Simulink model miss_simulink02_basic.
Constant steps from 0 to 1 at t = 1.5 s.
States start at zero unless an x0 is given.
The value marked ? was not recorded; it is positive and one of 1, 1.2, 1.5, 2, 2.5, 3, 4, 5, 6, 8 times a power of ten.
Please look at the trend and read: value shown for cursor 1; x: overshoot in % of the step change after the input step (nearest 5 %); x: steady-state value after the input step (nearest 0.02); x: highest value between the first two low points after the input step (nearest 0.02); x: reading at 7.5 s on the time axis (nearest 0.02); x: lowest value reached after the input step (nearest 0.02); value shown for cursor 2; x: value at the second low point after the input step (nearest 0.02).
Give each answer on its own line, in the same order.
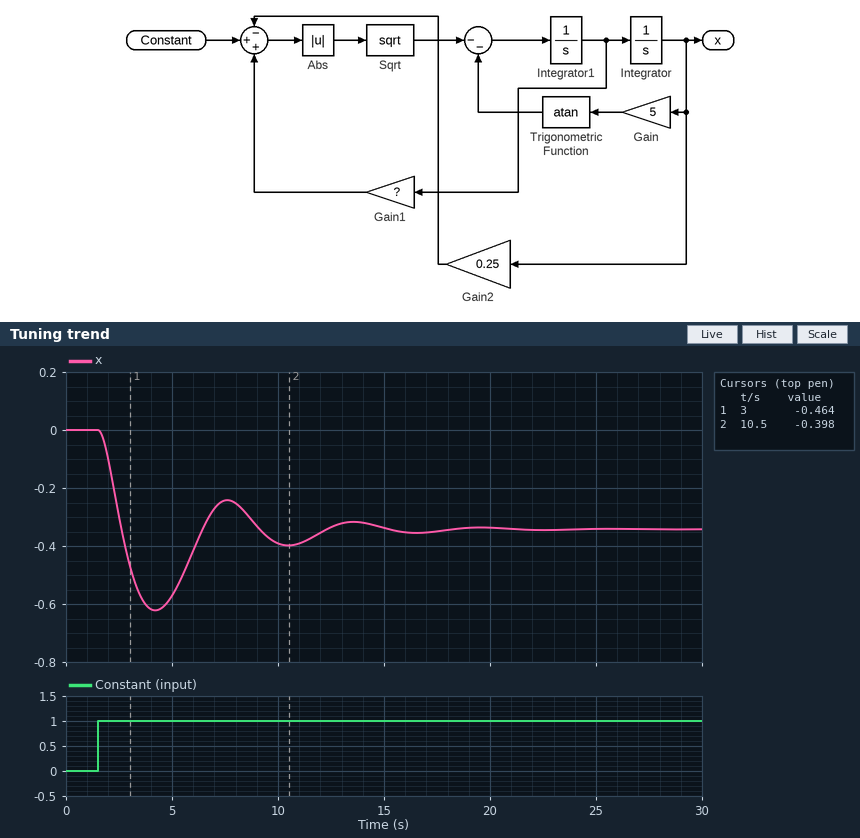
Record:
-0.464
80 %
-0.34
-0.24
-0.24
-0.62
-0.398
-0.40
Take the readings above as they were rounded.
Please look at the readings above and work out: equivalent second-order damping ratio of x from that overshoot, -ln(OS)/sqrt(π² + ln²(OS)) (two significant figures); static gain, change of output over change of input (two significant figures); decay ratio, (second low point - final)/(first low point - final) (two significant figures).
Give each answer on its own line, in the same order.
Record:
0.071
-0.34
0.21
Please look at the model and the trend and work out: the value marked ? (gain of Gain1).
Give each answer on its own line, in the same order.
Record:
1
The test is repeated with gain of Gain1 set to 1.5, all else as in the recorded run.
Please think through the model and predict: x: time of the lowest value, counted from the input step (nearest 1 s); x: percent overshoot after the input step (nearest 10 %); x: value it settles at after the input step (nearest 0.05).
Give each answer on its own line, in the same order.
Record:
3 s
50 %
-0.35
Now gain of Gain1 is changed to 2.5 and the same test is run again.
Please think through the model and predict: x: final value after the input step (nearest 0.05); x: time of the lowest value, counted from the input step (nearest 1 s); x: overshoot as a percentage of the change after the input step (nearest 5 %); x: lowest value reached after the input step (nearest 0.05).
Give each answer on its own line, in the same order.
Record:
-0.35
3 s
20 %
-0.40
